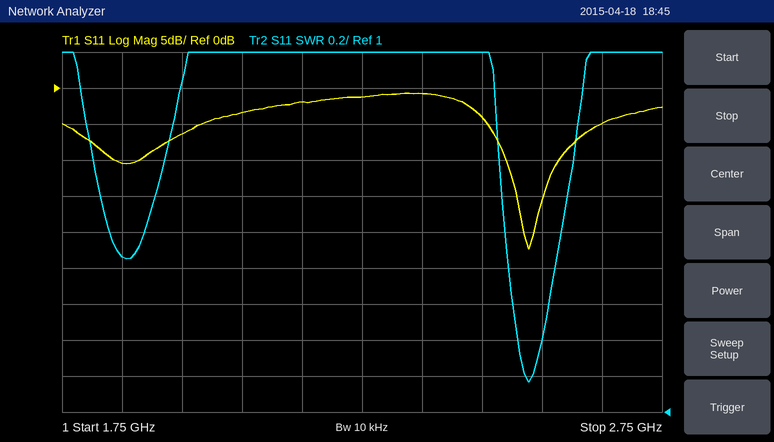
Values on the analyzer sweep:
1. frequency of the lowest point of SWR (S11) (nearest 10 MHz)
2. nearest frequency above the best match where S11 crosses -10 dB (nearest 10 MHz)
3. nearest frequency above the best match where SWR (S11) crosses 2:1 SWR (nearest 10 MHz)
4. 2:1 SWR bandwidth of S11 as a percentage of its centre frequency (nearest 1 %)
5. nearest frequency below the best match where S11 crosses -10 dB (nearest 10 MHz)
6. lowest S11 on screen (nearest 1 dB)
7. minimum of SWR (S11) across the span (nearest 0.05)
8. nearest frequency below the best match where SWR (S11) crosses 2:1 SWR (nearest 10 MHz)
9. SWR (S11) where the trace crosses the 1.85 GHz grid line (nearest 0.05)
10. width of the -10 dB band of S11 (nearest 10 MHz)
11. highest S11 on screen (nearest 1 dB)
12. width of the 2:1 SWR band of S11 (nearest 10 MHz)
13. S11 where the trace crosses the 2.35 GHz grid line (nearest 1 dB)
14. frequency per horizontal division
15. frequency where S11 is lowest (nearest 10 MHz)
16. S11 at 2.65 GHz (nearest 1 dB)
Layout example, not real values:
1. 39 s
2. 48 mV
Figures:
1. 2.53 GHz
2. 2.58 GHz
3. 2.58 GHz
4. 4 %
5. 2.49 GHz
6. -22 dB
7. 1.15
8. 2.49 GHz
9. 1.85
10. 90 MHz
11. -1 dB
12. 90 MHz
13. -1 dB
14. 100 MHz
15. 2.53 GHz
16. -5 dB
